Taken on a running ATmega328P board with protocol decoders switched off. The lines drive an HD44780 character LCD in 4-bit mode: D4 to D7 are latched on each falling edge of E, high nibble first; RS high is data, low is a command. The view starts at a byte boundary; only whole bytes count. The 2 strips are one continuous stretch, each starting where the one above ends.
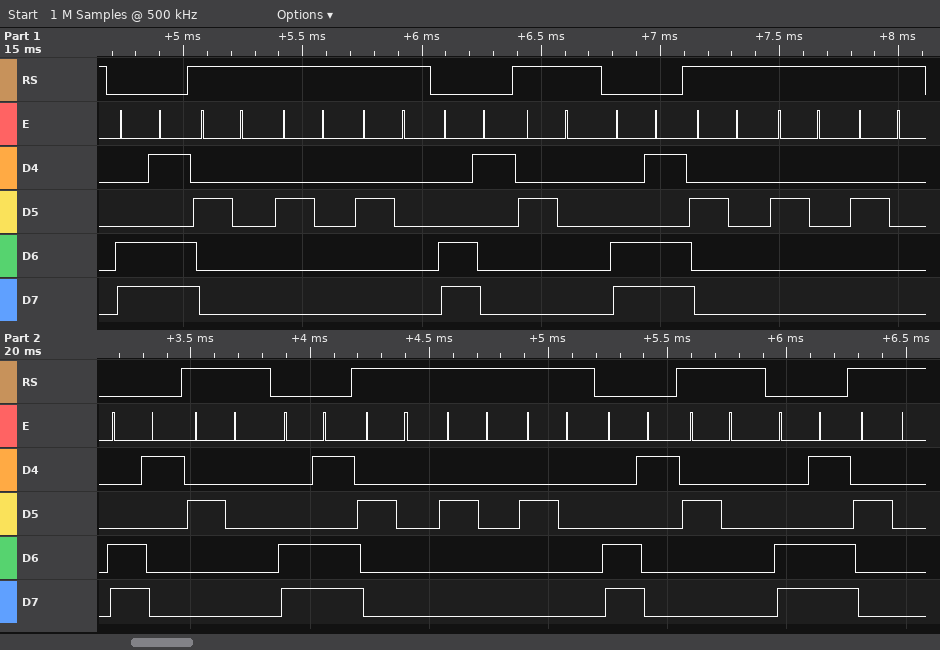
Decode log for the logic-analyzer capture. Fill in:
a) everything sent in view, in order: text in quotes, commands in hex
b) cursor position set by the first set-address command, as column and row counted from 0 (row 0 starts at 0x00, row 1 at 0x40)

0xCD "   " 0xC1 " " 0xCD "   " 0xC1 " " 0xCD "   " 0xC1 " " 0xCD " "
column 13, row 1
